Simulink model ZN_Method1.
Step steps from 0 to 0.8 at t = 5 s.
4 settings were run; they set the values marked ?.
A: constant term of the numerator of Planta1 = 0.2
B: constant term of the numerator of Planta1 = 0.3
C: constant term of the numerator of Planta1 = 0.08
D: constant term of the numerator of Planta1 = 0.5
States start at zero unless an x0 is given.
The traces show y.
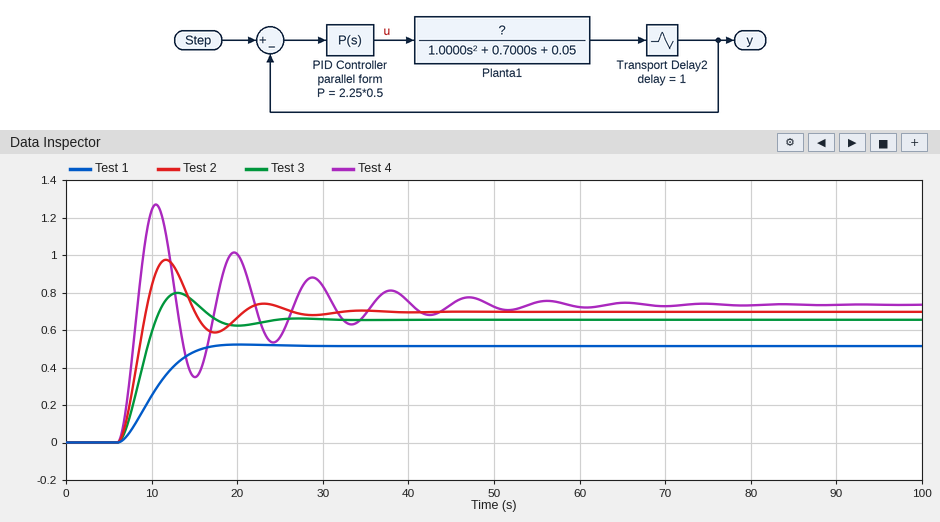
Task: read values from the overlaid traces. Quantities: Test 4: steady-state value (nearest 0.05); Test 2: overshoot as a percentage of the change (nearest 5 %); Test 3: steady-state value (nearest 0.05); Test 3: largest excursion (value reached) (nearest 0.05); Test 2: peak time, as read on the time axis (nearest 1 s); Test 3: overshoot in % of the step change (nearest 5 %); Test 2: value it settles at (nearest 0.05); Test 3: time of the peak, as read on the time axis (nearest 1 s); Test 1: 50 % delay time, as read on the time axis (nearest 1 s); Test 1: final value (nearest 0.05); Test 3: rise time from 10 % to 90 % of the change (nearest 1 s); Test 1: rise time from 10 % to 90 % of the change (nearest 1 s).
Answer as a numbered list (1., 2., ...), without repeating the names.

1. 0.75
2. 40 %
3. 0.65
4. 0.80
5. 12 s
6. 20 %
7. 0.70
8. 13 s
9. 10 s
10. 0.50
11. 3 s
12. 7 s
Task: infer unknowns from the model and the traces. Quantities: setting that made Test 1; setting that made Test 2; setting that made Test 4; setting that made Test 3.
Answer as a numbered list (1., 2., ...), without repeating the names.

1. C
2. B
3. D
4. A
